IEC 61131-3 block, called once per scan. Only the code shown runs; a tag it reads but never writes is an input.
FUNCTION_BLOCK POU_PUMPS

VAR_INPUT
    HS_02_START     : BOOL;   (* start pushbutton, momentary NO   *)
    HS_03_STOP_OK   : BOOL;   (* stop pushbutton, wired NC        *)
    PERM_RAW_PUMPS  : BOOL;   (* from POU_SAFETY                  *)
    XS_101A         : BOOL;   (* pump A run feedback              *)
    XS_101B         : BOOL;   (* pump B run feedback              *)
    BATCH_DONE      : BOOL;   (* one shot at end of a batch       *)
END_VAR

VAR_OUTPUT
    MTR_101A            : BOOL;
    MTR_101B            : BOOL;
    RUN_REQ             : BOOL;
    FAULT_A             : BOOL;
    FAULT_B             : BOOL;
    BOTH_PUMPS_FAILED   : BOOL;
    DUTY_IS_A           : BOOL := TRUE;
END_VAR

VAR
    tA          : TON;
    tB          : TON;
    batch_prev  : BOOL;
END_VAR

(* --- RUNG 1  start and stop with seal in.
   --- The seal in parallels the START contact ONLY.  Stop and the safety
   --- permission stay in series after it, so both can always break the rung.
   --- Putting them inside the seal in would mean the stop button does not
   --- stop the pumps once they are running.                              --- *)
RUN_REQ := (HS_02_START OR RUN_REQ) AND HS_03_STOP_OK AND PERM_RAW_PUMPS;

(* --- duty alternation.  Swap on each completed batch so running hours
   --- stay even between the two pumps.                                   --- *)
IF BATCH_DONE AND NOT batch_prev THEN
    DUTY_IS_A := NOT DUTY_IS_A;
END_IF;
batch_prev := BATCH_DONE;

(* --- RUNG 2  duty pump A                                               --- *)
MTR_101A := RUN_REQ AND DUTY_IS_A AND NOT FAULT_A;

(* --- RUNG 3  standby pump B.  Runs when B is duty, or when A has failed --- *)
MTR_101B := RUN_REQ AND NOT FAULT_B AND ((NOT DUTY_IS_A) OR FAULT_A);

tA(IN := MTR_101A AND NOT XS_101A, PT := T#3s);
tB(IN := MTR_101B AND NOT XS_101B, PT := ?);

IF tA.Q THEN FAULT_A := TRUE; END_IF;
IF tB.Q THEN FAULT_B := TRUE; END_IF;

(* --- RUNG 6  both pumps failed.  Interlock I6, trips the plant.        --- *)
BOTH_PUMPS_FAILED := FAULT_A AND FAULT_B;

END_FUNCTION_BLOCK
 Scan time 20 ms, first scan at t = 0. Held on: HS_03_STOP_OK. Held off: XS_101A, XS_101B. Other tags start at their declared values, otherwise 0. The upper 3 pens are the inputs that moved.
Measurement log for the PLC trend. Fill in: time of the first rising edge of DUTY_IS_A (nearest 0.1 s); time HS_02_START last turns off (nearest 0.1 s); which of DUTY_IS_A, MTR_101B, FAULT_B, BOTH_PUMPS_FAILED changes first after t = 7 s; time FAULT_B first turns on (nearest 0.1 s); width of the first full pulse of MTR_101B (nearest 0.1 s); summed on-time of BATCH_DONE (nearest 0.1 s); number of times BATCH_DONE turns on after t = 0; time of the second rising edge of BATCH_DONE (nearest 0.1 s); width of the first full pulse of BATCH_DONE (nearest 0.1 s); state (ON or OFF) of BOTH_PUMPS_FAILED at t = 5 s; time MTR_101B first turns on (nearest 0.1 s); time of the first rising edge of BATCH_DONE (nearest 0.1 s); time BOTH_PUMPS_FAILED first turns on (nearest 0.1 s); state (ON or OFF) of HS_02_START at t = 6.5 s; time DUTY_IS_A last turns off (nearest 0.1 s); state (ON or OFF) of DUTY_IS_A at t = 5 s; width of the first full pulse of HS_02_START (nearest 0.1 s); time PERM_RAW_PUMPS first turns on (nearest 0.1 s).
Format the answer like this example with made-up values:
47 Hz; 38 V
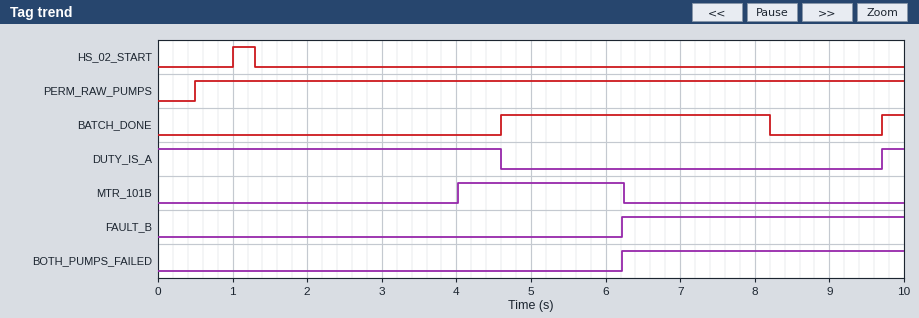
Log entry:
9.7 s; 1.3 s; DUTY_IS_A; 6.2 s; 2.2 s; 3.9 s; 2; 9.7 s; 3.6 s; OFF; 4.0 s; 4.6 s; 6.2 s; OFF; 4.6 s; OFF; 0.3 s; 0.5 s
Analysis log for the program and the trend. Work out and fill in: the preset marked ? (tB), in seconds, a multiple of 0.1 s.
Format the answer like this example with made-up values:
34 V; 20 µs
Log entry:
2.2 s
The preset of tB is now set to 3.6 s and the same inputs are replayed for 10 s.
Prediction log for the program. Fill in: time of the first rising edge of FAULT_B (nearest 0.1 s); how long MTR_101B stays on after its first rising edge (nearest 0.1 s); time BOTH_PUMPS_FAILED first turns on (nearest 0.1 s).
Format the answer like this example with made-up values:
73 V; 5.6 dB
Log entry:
7.6 s; 3.6 s; 7.6 s
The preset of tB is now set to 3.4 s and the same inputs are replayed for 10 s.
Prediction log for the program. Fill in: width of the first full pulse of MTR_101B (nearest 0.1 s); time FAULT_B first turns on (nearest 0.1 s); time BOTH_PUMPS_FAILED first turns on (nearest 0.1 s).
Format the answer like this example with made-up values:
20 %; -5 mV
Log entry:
3.4 s; 7.4 s; 7.4 s
